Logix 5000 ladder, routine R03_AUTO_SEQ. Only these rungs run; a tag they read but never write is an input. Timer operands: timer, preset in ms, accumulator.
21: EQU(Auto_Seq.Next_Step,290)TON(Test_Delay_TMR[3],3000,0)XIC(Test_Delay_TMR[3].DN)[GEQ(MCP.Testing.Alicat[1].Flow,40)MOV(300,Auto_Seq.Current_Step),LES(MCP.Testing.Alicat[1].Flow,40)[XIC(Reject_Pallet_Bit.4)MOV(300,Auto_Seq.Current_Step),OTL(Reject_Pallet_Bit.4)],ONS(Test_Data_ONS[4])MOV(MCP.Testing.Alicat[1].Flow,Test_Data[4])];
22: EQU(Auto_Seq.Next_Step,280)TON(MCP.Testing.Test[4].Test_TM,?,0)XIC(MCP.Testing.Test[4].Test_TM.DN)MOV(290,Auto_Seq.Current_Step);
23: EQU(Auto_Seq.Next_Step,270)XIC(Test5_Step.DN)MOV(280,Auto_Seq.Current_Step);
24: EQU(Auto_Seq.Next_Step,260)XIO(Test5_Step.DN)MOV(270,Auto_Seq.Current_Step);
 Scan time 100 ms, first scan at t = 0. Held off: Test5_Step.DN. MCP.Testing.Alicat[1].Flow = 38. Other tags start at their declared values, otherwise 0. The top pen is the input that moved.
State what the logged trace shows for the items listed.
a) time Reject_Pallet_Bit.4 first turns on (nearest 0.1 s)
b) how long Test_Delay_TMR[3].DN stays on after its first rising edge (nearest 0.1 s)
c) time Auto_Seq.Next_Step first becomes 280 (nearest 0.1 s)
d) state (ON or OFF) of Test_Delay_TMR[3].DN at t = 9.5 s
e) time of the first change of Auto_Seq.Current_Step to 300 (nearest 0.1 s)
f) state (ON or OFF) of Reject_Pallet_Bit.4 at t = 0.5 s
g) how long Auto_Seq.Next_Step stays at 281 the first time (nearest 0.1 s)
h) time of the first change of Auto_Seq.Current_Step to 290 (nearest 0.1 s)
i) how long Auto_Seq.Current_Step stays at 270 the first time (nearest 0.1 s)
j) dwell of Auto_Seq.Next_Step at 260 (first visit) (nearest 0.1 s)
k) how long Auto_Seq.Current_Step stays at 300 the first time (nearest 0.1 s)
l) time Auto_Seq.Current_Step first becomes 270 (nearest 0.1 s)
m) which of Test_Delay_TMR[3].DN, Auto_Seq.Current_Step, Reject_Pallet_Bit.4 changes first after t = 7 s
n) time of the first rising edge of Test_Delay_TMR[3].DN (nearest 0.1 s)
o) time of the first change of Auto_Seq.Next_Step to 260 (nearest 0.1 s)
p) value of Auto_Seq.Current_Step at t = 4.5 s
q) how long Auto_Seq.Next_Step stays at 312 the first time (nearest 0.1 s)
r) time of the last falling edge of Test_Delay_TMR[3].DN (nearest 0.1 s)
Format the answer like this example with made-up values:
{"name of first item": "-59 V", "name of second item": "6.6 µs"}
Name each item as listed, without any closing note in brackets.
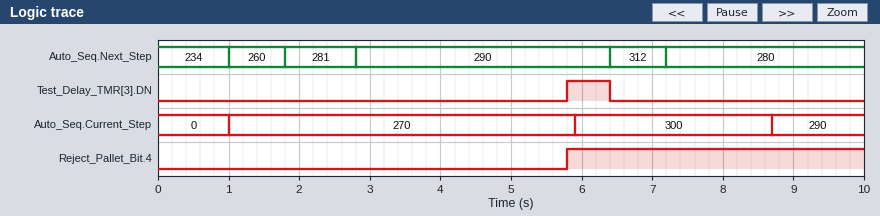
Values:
{"time Reject_Pallet_Bit.4 first turns on": "5.8 s", "how long Test_Delay_TMR[3].DN stays on after its first rising edge": "0.6 s", "time Auto_Seq.Next_Step first becomes 280": "7.2 s", "state (ON or OFF) of Test_Delay_TMR[3].DN at t = 9.5 s": "OFF", "time of the first change of Auto_Seq.Current_Step to 300": "5.9 s", "state (ON or OFF) of Reject_Pallet_Bit.4 at t = 0.5 s": "OFF", "how long Auto_Seq.Next_Step stays at 281 the first time": "1.0 s", "time of the first change of Auto_Seq.Current_Step to 290": "8.7 s", "how long Auto_Seq.Current_Step stays at 270 the first time": "4.9 s", "dwell of Auto_Seq.Next_Step at 260 (first visit)": "0.8 s", "how long Auto_Seq.Current_Step stays at 300 the first time": "2.8 s", "time Auto_Seq.Current_Step first becomes 270": "1.0 s", "which of Test_Delay_TMR[3].DN, Auto_Seq.Current_Step, Reject_Pallet_Bit.4 changes first after t = 7 s": "Auto_Seq.Current_Step", "time of the first rising edge of Test_Delay_TMR[3].DN": "5.8 s", "time of the first change of Auto_Seq.Next_Step to 260": "1.0 s", "value of Auto_Seq.Current_Step at t = 4.5 s": "270", "how long Auto_Seq.Next_Step stays at 312 the first time": "0.8 s", "time of the last falling edge of Test_Delay_TMR[3].DN": "6.4 s"}
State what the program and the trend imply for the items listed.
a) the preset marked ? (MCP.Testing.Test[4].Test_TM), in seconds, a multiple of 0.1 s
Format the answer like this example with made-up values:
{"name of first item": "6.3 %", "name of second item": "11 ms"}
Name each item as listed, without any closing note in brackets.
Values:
{"the preset marked ? (MCP.Testing.Test[4].Test_TM), in seconds, a multiple of 0.1 s": "1.5 s"}
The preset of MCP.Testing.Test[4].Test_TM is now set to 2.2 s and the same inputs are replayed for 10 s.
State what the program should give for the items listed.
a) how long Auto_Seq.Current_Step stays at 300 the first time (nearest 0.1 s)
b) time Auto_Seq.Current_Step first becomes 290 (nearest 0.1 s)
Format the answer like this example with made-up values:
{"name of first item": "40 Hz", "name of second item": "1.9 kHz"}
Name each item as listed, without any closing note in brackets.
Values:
{"how long Auto_Seq.Current_Step stays at 300 the first time": "3.5 s", "time Auto_Seq.Current_Step first becomes 290": "9.4 s"}
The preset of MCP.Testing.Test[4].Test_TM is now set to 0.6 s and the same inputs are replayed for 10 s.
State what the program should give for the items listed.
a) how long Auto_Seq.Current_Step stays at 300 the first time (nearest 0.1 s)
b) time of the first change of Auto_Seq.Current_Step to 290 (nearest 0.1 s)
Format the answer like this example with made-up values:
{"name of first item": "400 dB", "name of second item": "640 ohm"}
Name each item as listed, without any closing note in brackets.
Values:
{"how long Auto_Seq.Current_Step stays at 300 the first time": "1.9 s", "time of the first change of Auto_Seq.Current_Step to 290": "7.8 s"}
